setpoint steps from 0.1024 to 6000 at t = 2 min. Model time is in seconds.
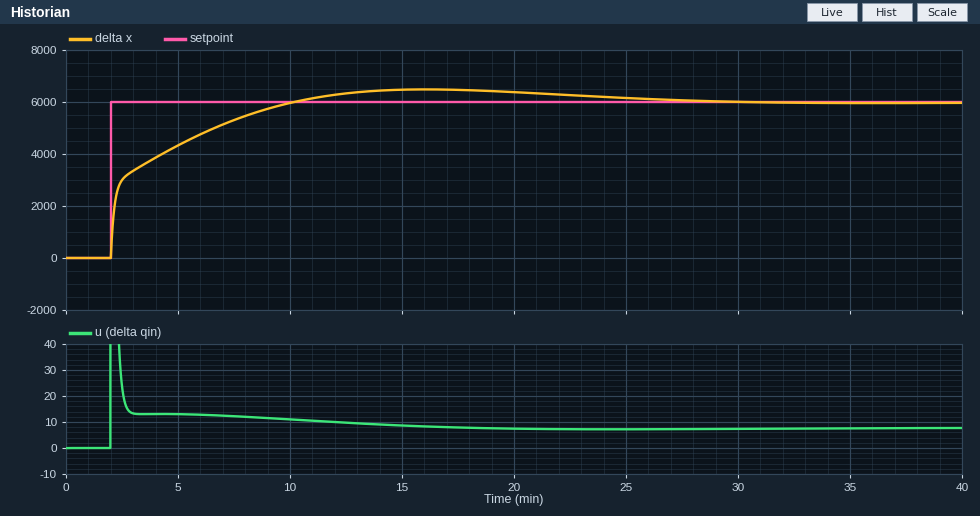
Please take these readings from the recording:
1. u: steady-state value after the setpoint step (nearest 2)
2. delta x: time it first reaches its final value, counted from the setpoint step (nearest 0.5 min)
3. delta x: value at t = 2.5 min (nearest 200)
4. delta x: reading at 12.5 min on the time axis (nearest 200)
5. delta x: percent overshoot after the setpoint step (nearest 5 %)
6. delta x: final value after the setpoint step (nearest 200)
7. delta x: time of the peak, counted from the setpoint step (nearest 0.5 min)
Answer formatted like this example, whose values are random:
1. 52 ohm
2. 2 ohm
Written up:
1. 8
2. 8.0 min
3. 3000
4. 6400
5. 10 %
6. 6000
7. 14.0 min
